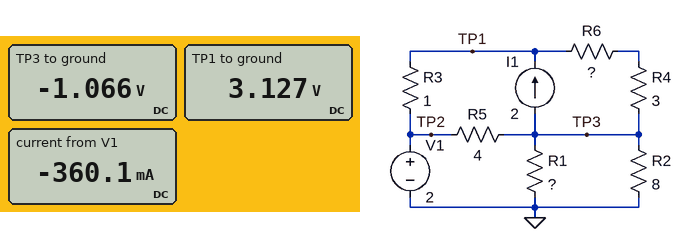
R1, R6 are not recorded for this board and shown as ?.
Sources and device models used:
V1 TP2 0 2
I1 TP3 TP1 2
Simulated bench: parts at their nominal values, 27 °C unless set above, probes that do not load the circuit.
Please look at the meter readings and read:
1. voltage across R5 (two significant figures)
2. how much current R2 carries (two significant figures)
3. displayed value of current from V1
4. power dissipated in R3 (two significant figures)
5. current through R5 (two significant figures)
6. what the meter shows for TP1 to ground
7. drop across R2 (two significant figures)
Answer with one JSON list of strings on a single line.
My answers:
["3.1 V", "130 mA", "-360.1 mA", "1.3 W", "770 mA", "3.127 V", "1.1 V"]
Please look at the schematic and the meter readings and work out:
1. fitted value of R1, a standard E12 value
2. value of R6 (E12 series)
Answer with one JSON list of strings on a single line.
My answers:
["4.7 Ω", "1.8 Ω"]
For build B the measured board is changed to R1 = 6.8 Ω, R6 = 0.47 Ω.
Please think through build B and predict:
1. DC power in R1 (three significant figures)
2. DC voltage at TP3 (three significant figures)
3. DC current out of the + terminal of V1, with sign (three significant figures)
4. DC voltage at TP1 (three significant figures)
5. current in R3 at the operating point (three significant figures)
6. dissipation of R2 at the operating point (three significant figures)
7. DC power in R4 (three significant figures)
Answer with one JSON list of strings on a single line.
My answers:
["96.8 mW", "-811 mV", "-221 mA", "2.92 V", "924 mA", "82.3 mW", "3.48 W"]
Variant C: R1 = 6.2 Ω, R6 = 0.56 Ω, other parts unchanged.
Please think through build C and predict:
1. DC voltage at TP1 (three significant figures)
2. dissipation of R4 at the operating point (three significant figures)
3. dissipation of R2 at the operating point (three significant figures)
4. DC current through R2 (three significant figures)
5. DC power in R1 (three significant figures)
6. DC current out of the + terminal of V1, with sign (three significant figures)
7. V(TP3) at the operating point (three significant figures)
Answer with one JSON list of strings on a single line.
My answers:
["2.94 V", "3.36 W", "84.9 mW", "103 mA", "110 mW", "-236 mA", "-824 mV"]
